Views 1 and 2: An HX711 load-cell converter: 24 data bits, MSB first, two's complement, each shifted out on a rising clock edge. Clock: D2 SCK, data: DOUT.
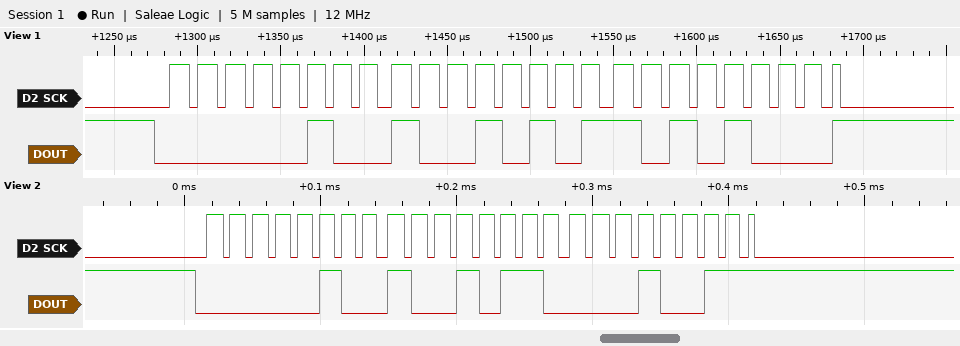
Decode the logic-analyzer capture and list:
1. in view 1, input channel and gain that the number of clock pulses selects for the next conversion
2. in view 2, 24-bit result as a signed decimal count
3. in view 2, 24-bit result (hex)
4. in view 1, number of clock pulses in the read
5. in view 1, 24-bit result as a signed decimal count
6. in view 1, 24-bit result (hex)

channel A, gain 128
300563
0x049613
25
300456
0x0495A8
